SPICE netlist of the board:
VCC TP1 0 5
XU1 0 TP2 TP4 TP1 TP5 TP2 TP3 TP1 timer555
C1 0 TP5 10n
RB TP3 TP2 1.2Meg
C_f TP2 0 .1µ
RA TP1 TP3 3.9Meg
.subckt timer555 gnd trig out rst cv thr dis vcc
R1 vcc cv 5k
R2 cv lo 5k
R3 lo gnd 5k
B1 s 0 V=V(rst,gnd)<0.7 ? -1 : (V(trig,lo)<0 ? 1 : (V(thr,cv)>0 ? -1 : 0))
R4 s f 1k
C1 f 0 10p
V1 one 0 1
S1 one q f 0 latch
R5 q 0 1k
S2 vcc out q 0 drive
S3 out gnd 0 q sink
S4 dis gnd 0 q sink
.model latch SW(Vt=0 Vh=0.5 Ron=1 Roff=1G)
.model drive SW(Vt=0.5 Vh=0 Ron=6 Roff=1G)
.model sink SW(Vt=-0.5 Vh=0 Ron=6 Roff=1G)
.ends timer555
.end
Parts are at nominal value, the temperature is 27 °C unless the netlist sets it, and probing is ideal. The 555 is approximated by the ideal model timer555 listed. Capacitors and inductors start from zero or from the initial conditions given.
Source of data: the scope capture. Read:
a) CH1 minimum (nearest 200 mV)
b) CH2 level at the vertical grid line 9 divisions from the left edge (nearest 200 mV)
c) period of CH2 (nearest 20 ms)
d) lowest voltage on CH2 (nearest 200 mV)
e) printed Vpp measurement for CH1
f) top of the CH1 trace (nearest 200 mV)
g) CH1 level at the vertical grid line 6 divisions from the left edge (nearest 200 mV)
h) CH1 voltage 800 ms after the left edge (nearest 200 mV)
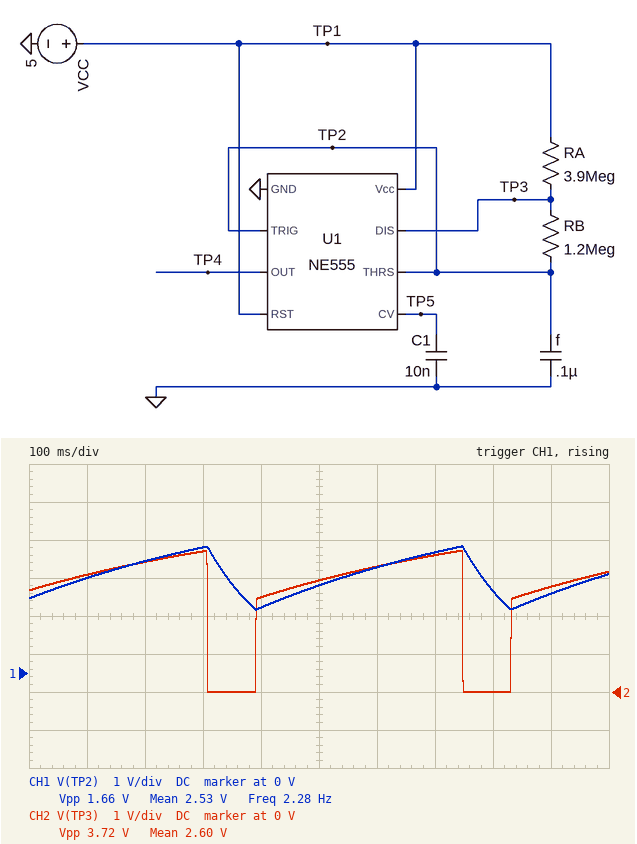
1.6 V
2.8 V
440 ms
0 V
1.66 V
3.4 V
2.8 V
2.2 V
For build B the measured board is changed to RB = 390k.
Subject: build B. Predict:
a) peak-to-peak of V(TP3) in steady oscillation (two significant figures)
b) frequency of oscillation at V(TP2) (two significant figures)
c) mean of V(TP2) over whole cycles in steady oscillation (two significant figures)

3.5 V
3.1 Hz
2.6 V
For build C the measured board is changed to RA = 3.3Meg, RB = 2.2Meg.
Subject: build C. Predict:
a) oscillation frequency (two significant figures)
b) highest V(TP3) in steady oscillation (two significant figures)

1.9 Hz
4.0 V
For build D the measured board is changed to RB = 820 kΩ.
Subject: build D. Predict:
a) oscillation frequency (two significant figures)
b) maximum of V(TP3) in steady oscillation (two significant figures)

2.6 Hz
3.6 V
